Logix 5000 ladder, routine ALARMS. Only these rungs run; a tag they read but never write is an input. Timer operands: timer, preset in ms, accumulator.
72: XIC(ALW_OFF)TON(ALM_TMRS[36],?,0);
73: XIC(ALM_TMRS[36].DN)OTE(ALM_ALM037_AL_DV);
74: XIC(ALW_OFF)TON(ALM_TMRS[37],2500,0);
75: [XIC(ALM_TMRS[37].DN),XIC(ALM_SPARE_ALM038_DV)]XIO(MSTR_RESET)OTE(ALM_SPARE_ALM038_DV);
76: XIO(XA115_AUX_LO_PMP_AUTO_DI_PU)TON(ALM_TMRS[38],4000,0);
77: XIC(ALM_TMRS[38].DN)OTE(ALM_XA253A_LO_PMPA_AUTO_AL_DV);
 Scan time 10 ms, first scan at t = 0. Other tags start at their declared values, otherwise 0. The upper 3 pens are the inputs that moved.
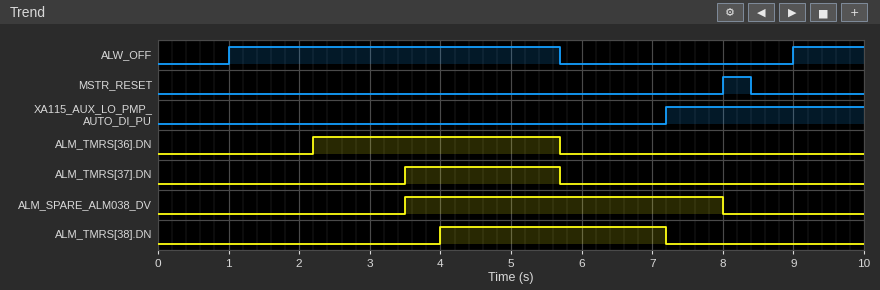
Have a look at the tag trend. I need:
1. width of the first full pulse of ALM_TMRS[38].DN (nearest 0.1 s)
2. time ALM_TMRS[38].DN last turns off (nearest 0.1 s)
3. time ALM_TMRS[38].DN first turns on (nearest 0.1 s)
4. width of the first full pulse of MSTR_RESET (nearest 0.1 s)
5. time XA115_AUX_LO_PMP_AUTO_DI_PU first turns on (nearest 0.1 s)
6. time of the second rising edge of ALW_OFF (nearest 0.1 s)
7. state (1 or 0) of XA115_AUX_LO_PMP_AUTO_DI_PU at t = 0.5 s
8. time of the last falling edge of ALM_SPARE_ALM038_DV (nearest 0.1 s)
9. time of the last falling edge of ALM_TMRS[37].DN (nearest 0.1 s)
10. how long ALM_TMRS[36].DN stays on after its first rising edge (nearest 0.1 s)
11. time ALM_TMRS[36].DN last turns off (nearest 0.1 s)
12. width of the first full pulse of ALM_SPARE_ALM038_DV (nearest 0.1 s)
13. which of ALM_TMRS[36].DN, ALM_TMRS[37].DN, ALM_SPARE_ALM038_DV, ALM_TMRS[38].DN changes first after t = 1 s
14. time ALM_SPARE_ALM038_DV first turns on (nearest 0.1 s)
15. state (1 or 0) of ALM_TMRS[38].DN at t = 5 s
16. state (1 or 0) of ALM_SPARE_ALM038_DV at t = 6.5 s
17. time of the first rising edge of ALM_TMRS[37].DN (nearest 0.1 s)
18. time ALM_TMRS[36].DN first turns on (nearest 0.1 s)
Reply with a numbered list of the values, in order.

1. 3.2 s
2. 7.2 s
3. 4.0 s
4. 0.4 s
5. 7.2 s
6. 9.0 s
7. 0
8. 8.0 s
9. 5.7 s
10. 3.5 s
11. 5.7 s
12. 4.5 s
13. ALM_TMRS[36].DN
14. 3.5 s
15. 1
16. 1
17. 3.5 s
18. 2.2 s
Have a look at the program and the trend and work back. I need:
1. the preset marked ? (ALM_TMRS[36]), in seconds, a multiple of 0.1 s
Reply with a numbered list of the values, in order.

1. 1.2 s
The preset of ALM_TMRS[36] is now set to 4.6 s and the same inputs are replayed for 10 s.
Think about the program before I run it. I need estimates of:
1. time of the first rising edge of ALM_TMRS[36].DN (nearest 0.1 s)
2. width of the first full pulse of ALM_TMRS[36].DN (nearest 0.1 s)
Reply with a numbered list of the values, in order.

1. 5.6 s
2. 0.1 s
